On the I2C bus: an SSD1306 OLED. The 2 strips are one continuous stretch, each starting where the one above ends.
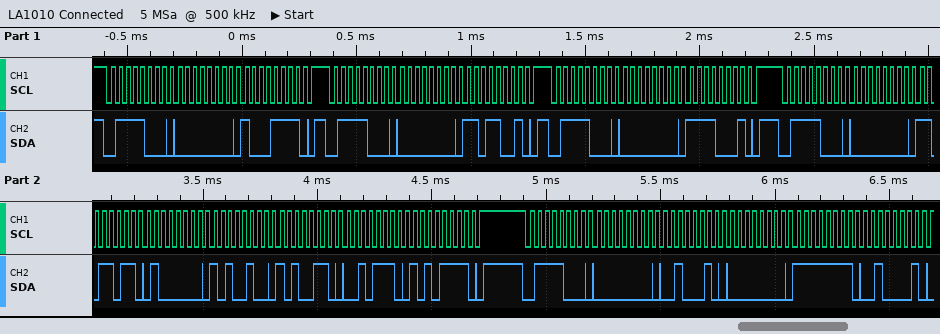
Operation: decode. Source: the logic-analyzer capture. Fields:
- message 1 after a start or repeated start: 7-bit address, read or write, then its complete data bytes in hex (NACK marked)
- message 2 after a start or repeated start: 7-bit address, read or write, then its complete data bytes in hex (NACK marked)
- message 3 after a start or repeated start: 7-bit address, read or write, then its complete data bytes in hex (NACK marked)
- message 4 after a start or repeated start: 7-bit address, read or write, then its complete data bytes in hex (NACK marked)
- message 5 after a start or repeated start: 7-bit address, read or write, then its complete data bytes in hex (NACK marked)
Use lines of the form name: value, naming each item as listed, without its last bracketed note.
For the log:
message 1 after a start or repeated start: 7-bit address, read or write, then its complete data bytes in hex: 0x3C write: 00 8F
message 2 after a start or repeated start: 7-bit address, read or write, then its complete data bytes in hex: 0x3C write: 00 D9
message 3 after a start or repeated start: 7-bit address, read or write, then its complete data bytes in hex: 0x3C write: 00 F1
message 4 after a start or repeated start: 7-bit address, read or write, then its complete data bytes in hex: 0x3C write: 00 DB 40 A4 A6 2E AF
message 5 after a start or repeated start: 7-bit address, read or write, then its complete data bytes in hex: 0x3C write: 00 22 00 FF 21
